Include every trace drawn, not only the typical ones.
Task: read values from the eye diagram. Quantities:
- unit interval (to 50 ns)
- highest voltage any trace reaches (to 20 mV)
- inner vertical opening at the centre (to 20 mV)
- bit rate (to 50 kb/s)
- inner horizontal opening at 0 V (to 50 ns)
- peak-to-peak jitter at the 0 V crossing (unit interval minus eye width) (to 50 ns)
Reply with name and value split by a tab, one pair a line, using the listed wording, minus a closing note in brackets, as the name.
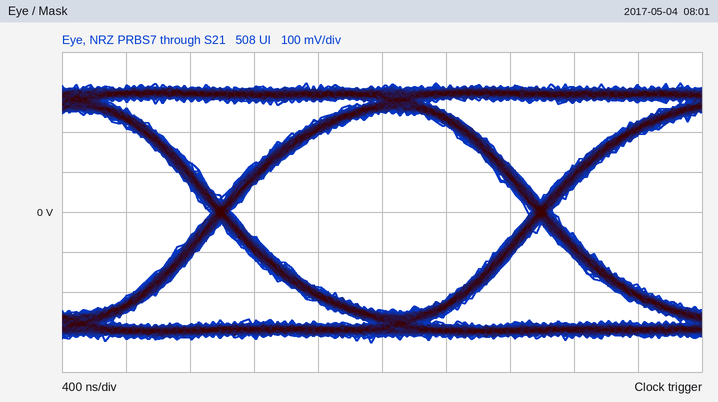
unit interval	2.00 µs
highest voltage any trace reaches	320 mV
inner vertical opening at the centre	500 mV
bit rate	500 kb/s
inner horizontal opening at 0 V	1.85 µs
peak-to-peak jitter at the 0 V crossing (unit interval minus eye width)	150 ns
